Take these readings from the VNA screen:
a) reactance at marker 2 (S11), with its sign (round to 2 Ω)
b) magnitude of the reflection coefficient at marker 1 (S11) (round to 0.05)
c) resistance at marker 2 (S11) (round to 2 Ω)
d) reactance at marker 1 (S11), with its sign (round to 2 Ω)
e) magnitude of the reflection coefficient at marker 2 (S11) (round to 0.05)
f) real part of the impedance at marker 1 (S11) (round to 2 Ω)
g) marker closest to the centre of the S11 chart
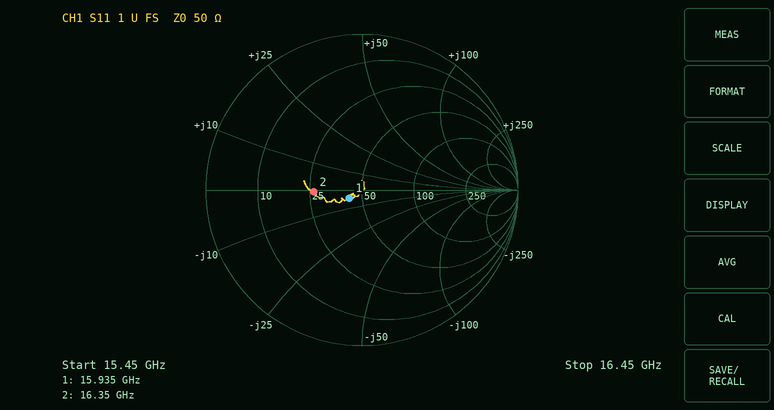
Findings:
0 Ω
0.10
26 Ω
-4 Ω
0.30
42 Ω
marker 1
